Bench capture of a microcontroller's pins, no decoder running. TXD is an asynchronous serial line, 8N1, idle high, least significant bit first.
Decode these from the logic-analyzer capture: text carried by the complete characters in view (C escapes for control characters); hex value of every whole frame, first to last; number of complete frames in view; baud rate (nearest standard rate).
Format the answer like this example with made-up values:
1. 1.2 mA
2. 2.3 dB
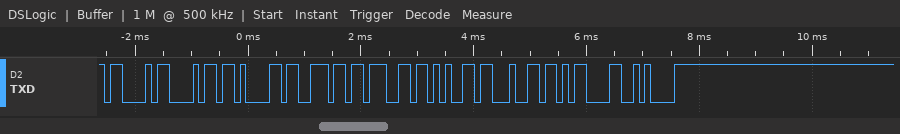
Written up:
1. "Changed\r\n"
2. 0x43 0x68 0x61 0x6E 0x67 0x65 0x64 0x0D 0x0A
3. 9
4. 9600 baud
